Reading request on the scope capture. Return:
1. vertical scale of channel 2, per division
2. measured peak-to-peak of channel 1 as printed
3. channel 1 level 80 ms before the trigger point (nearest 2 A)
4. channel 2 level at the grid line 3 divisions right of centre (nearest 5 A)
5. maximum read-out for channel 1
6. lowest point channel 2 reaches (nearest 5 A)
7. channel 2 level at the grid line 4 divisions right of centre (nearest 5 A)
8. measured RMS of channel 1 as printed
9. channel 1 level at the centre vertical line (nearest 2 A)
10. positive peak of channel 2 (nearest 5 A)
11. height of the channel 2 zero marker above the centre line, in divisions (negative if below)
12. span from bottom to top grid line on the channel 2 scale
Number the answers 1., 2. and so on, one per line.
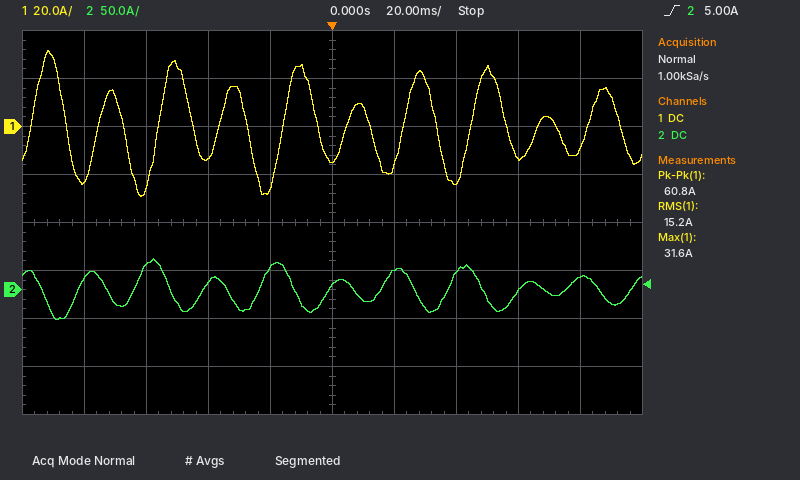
1. 50 A
2. 60.8 A
3. -22 A
4. 0 A
5. 31.6 A
6. -30 A
7. 15 A
8. 15.2 A
9. -14 A
10. 30 A
11. -1.4 div
12. 400 A
